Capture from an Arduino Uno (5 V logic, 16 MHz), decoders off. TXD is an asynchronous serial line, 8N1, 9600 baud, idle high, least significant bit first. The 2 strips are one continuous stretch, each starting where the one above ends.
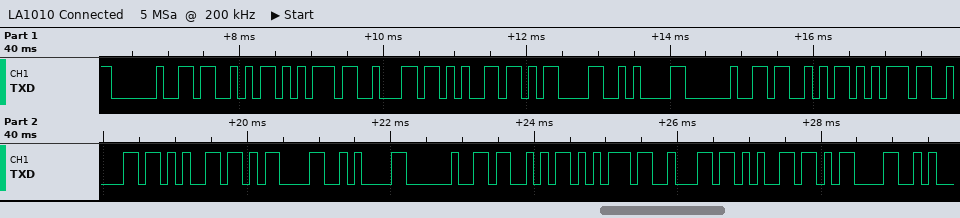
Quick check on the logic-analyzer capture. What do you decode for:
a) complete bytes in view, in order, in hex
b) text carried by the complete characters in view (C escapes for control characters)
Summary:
20 53 75 62 65 0D 0A 20 53 75 62 65 0D 0A 20 53 75 62 65 0D
" Sube\r\n Sube\r\n Sube\r"
